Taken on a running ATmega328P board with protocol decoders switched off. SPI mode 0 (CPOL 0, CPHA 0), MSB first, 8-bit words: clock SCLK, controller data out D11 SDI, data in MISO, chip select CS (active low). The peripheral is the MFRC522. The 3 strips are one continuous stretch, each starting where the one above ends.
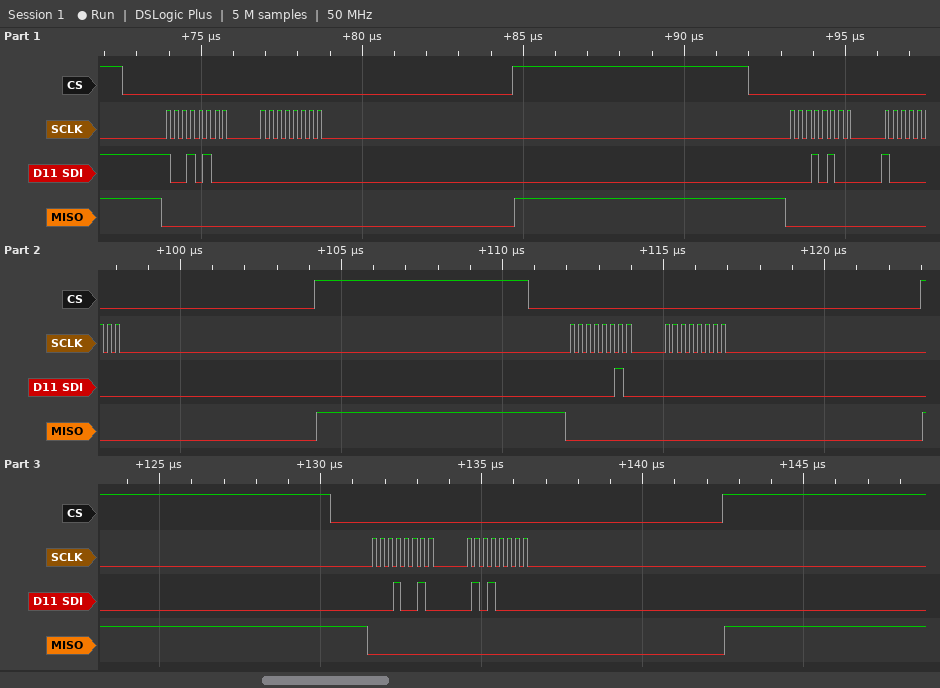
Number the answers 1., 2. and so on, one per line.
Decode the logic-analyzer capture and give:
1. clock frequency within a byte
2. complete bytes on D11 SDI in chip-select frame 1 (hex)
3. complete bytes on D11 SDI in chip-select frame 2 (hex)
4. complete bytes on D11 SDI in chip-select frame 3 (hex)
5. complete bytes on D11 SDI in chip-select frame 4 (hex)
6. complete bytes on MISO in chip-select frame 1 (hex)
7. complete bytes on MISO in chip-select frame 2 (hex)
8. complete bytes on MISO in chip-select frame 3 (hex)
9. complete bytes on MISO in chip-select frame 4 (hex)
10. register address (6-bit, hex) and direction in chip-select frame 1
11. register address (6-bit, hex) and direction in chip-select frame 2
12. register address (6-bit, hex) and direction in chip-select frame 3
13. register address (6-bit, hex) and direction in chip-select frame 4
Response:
1. 4 MHz
2. 94 00
3. 14 80
4. 02 00
5. 12 50
6. 00 00
7. 00 00
8. 00 00
9. 00 00
10. 0x0A read
11. 0x0A write
12. 0x01 write
13. 0x09 write
